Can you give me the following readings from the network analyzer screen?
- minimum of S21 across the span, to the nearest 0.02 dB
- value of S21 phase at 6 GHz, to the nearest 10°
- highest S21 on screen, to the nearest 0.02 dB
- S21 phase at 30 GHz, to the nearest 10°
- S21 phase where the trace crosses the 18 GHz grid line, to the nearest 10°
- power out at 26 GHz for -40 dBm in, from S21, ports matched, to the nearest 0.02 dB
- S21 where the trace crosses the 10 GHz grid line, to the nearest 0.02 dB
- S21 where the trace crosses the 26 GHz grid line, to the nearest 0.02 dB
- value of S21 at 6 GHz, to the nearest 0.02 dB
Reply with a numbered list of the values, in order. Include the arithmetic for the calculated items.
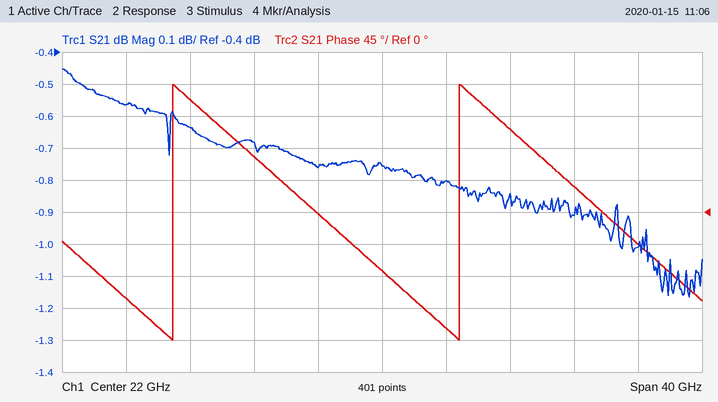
1. -1.16 dB
2. -120°
3. -0.46 dB
4. 120°
5. 0°
6. -40 dBm + (-0.80 dB) = -40.80 dBm
7. -0.64 dB
8. -0.80 dB
9. -0.56 dB
